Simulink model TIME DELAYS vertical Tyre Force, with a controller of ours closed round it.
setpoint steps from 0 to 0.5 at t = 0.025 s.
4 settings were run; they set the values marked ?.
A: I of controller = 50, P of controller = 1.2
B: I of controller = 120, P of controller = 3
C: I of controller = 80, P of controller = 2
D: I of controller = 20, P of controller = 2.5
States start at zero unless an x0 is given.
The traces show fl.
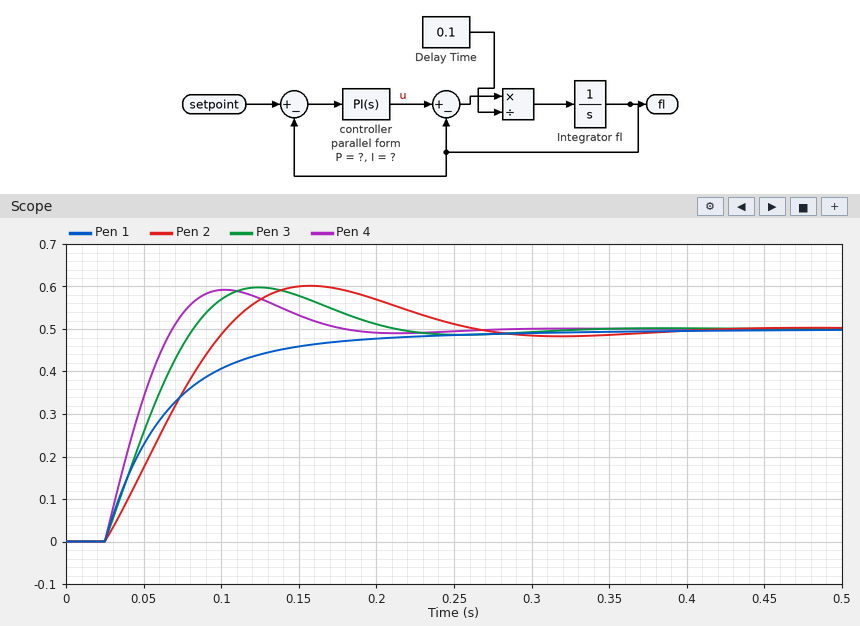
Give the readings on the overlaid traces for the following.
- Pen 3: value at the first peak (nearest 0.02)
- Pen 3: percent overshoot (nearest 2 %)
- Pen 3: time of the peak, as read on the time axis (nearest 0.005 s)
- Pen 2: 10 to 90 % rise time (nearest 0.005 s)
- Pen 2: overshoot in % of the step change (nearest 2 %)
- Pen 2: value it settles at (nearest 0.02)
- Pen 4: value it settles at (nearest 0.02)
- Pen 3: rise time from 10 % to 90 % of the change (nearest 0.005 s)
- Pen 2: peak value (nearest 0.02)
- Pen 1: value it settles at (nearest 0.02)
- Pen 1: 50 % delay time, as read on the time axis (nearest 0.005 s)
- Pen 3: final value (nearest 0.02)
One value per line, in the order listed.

0.60
20 %
0.125 s
0.060 s
20 %
0.50
0.50
0.045 s
0.60
0.50
0.055 s
0.50
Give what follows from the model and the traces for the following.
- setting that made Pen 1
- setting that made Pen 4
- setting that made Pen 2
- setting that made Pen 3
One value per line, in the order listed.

D
B
A
C
